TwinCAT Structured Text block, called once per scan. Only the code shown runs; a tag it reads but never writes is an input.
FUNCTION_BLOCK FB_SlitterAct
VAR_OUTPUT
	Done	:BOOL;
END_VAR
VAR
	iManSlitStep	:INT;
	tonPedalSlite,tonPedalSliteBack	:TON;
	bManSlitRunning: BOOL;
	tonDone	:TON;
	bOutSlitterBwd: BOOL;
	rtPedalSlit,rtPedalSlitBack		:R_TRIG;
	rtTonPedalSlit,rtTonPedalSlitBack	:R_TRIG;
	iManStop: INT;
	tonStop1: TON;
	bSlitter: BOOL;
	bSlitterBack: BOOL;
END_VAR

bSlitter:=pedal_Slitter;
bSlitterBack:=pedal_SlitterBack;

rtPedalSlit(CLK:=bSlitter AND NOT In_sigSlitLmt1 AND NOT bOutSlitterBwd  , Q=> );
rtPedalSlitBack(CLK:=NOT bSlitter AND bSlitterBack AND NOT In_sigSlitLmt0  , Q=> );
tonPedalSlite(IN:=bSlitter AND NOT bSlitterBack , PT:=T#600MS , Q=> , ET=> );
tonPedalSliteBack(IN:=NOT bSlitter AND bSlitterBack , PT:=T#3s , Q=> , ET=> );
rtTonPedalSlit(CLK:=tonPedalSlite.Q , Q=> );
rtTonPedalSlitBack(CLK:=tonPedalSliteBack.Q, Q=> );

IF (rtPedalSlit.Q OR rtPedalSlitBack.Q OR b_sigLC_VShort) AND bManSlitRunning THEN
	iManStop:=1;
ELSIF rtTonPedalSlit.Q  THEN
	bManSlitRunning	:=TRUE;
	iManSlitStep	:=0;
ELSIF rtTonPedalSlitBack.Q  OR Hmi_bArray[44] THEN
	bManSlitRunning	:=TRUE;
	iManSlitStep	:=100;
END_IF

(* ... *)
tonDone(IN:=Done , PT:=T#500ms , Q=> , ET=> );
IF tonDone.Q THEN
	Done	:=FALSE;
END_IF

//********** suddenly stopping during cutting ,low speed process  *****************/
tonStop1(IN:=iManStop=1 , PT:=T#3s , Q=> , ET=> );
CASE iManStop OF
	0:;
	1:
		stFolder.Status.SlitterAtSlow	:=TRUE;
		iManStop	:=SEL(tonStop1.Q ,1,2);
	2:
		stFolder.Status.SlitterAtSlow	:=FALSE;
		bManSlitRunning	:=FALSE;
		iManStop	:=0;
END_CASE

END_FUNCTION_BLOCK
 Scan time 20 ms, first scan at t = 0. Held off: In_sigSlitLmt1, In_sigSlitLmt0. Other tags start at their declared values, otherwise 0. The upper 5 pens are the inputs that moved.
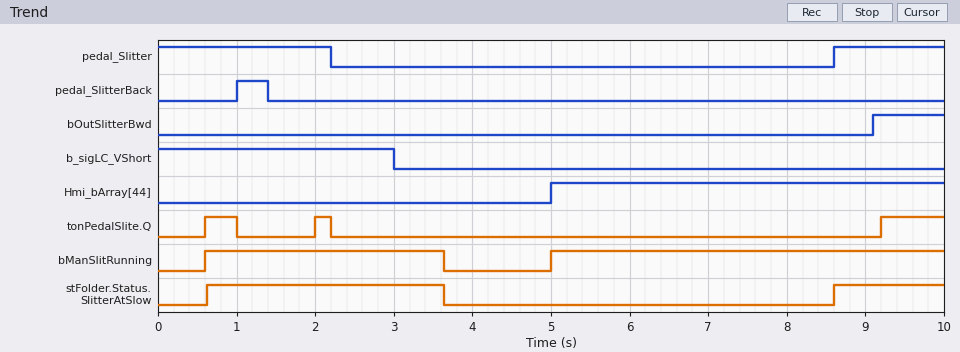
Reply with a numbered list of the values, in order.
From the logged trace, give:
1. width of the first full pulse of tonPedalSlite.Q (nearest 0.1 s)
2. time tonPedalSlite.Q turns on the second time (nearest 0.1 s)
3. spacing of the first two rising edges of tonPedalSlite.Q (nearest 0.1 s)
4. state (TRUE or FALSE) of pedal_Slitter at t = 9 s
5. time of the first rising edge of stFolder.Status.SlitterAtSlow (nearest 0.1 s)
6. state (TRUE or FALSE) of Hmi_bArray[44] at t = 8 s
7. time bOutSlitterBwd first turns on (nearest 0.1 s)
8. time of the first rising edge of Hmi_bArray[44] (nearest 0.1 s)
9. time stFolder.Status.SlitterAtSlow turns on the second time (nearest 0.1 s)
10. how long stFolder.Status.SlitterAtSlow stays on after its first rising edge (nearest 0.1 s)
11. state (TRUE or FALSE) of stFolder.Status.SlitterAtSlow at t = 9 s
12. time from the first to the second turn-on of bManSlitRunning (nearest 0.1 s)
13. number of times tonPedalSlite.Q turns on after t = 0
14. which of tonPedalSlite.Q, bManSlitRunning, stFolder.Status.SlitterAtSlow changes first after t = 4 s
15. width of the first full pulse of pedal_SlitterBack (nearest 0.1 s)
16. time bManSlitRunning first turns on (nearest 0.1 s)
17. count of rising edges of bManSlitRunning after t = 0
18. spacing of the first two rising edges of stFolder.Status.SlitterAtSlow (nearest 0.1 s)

1. 0.4 s
2. 2.0 s
3. 1.4 s
4. TRUE
5. 0.6 s
6. TRUE
7. 9.1 s
8. 5.0 s
9. 8.6 s
10. 3.0 s
11. TRUE
12. 4.4 s
13. 3
14. bManSlitRunning
15. 0.4 s
16. 0.6 s
17. 2
18. 8.0 s
